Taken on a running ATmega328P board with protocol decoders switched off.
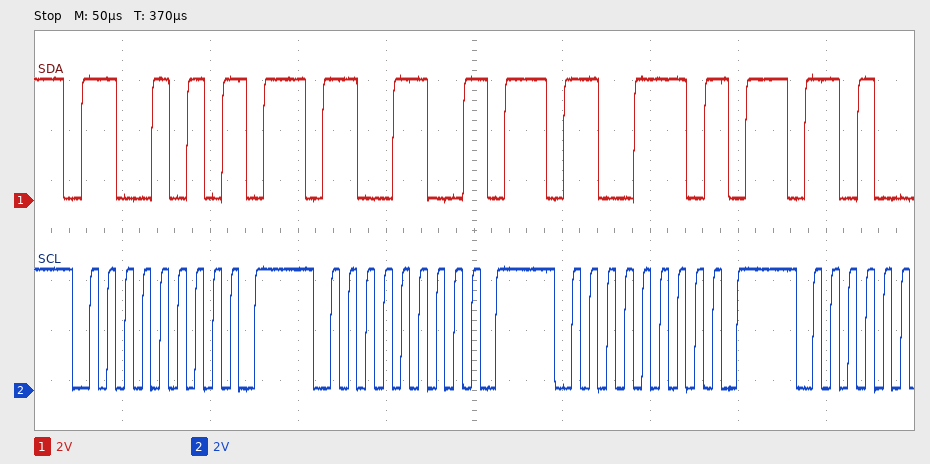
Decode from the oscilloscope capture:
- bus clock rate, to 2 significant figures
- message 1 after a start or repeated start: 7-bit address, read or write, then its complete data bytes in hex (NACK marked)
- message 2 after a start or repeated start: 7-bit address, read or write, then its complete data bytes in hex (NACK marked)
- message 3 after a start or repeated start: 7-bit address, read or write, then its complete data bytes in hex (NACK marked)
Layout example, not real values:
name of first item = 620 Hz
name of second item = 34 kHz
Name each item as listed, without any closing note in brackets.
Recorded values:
bus clock rate, to 2 significant figures = 100 kHz
message 1 after a start or repeated start: 7-bit address, read or write, then its complete data bytes in hex = 0x65 write NACK
message 2 after a start or repeated start: 7-bit address, read or write, then its complete data bytes in hex = 0x66 write NACK
message 3 after a start or repeated start: 7-bit address, read or write, then its complete data bytes in hex = 0x67 write NACK
